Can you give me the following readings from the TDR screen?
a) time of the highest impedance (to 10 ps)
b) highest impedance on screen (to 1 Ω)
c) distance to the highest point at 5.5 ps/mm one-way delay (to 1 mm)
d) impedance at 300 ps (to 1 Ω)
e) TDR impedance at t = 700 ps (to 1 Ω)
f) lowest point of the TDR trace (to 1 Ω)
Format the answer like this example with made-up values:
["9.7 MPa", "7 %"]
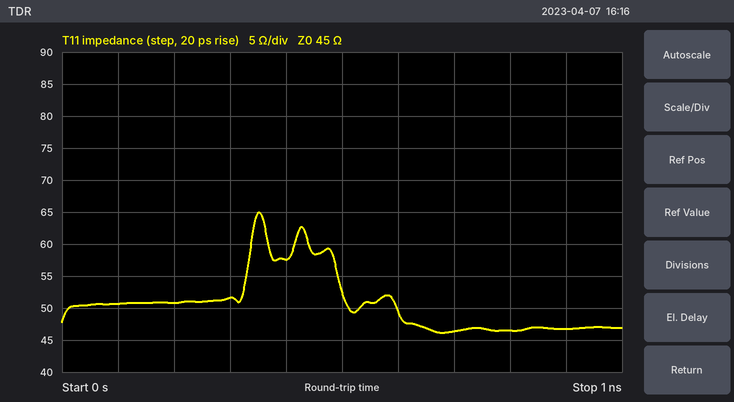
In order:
["350 ps", "65 Ω", "32 mm", "52 Ω", "46 Ω", "46 Ω"]
